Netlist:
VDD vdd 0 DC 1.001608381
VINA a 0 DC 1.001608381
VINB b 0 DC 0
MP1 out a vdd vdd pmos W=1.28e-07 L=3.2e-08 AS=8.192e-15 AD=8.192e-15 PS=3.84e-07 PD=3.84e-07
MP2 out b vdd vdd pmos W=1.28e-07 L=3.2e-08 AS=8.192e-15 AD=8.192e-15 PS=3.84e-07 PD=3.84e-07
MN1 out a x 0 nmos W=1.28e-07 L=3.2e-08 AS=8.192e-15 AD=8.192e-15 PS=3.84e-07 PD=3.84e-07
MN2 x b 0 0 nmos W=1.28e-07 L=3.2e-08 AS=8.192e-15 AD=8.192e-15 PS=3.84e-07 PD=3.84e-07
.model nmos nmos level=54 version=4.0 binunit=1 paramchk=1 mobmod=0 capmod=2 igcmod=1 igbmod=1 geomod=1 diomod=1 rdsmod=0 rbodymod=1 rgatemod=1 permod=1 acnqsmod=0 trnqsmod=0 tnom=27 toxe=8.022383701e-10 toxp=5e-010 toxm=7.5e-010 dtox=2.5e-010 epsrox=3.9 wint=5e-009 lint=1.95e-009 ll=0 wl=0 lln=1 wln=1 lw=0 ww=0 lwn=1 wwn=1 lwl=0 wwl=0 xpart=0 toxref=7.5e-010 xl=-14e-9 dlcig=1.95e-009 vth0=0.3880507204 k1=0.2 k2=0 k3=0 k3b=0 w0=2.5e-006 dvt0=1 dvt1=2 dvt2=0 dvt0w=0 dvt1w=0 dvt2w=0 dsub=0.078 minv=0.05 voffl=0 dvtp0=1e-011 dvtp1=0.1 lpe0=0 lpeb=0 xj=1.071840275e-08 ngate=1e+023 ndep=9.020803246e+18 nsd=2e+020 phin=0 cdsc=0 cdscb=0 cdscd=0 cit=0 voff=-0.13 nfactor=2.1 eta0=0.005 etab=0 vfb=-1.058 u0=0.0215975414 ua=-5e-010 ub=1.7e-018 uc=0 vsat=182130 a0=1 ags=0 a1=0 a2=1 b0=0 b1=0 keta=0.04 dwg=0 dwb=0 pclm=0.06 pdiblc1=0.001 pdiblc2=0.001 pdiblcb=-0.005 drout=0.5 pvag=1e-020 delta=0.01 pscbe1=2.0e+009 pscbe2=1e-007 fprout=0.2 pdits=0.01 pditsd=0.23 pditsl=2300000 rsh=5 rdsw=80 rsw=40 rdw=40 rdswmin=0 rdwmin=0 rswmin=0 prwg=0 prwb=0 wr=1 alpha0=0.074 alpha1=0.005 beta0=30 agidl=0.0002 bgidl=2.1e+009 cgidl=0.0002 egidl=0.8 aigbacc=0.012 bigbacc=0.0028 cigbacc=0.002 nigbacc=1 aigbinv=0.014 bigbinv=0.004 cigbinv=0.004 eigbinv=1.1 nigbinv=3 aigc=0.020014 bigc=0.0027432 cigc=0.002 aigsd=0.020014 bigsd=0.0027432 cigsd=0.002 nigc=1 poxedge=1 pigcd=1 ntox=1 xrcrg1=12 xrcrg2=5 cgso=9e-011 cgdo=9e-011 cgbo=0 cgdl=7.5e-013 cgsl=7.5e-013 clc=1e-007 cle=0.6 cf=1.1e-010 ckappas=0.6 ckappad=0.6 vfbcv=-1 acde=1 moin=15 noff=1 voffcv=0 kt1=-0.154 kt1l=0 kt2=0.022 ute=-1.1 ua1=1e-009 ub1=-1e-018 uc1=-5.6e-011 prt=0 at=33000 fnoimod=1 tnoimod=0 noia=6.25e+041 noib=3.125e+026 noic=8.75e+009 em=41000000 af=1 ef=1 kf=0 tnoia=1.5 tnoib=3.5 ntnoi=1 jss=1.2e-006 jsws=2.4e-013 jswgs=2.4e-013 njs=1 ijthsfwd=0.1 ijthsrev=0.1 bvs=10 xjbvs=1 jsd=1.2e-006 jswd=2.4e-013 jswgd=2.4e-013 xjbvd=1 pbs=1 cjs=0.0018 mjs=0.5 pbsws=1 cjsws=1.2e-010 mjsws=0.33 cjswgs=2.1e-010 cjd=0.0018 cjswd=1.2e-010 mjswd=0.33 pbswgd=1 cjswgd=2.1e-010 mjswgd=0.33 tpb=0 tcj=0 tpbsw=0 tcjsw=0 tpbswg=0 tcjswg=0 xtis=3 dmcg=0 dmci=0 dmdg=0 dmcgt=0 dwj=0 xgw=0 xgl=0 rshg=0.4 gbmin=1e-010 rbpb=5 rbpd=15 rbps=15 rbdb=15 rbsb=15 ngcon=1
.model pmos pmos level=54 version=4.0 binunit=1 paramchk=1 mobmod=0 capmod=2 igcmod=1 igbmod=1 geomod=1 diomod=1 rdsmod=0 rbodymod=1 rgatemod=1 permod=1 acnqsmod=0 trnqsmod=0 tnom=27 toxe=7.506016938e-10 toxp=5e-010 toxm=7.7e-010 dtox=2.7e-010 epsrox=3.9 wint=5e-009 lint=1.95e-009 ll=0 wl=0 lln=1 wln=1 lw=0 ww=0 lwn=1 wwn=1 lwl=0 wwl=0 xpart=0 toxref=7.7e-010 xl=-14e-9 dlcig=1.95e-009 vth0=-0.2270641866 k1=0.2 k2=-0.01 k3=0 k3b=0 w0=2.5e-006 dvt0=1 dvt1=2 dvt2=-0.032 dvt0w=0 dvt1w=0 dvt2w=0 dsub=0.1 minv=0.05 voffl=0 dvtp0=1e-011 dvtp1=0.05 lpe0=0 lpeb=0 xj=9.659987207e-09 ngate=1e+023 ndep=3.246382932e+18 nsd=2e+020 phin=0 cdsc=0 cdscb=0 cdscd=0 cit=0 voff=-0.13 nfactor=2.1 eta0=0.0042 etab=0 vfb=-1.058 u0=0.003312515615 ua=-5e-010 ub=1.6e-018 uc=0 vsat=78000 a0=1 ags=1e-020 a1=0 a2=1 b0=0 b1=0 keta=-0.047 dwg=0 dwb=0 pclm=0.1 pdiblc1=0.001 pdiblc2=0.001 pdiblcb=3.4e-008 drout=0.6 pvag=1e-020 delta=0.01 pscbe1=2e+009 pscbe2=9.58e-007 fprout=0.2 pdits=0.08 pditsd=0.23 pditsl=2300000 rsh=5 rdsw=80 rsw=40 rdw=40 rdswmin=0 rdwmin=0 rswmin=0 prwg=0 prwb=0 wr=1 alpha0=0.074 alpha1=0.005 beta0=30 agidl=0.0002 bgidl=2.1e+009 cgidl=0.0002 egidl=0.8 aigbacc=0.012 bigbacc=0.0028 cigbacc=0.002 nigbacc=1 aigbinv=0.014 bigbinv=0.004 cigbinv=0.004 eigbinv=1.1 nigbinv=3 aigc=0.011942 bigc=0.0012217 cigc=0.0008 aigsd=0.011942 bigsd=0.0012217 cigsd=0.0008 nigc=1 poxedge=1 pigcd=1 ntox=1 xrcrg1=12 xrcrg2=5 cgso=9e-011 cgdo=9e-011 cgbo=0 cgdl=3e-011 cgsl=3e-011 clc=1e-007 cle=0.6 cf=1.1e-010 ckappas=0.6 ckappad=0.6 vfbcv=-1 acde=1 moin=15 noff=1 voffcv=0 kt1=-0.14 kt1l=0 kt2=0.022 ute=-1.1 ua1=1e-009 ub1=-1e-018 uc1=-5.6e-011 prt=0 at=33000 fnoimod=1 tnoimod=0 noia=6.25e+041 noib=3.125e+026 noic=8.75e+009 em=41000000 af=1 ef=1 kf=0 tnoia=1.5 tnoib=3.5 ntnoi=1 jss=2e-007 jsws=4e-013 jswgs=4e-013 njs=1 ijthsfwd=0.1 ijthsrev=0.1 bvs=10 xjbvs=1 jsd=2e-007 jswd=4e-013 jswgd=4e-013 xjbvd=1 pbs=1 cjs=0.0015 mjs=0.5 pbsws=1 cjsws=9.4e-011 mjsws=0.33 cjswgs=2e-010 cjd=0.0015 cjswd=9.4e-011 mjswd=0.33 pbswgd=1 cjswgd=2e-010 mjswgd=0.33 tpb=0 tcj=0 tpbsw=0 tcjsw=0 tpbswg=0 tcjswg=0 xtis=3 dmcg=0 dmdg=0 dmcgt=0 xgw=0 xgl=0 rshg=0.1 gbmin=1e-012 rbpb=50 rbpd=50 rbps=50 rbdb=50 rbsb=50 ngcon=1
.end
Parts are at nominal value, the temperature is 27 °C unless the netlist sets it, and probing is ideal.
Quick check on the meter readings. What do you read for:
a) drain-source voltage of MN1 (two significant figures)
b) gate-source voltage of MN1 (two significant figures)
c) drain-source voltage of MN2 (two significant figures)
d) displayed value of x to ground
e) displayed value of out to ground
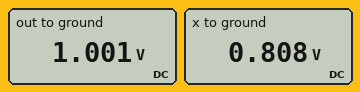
190 mV
190 mV
810 mV
0.808 V
1.001 V
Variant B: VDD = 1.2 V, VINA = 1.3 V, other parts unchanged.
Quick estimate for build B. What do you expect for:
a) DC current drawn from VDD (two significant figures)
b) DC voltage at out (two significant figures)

300 nA
1.2 V
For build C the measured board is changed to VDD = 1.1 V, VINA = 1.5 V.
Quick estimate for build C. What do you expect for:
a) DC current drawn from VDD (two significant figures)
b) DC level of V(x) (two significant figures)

170 nA
1.1 V
